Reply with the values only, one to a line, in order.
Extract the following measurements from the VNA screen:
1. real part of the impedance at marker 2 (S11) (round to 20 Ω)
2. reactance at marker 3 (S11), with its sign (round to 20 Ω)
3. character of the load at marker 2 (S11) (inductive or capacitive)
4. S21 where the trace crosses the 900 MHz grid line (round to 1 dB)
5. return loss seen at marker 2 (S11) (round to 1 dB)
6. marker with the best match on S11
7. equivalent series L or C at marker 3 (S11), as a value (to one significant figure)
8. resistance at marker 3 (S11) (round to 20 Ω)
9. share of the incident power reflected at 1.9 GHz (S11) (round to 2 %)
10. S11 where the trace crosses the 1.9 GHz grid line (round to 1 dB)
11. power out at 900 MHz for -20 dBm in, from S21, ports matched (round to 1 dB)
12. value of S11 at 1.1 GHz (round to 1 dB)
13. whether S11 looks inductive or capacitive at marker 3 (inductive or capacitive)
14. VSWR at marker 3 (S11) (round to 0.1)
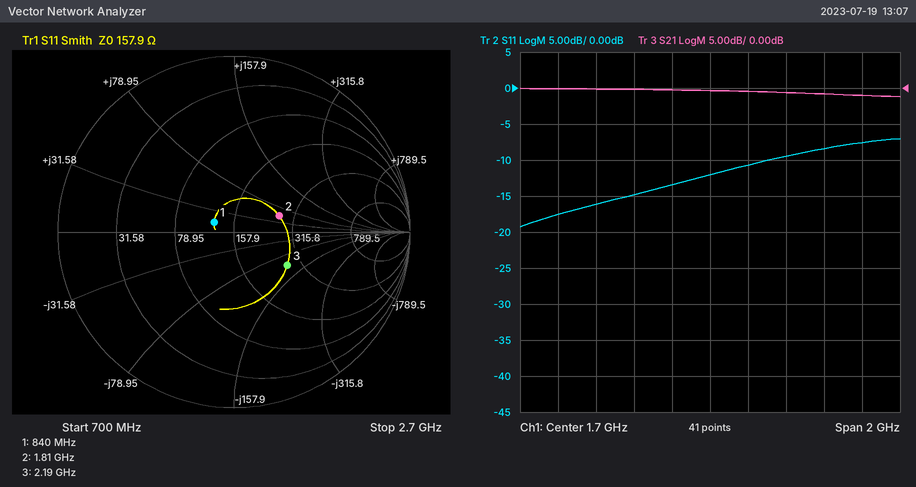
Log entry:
260 Ω
-120 Ω
inductive
0 dB
11 dB
marker 1
600 fF
260 Ω
8 %
-11 dB
-20 dBm
-16 dB
capacitive
2.1
